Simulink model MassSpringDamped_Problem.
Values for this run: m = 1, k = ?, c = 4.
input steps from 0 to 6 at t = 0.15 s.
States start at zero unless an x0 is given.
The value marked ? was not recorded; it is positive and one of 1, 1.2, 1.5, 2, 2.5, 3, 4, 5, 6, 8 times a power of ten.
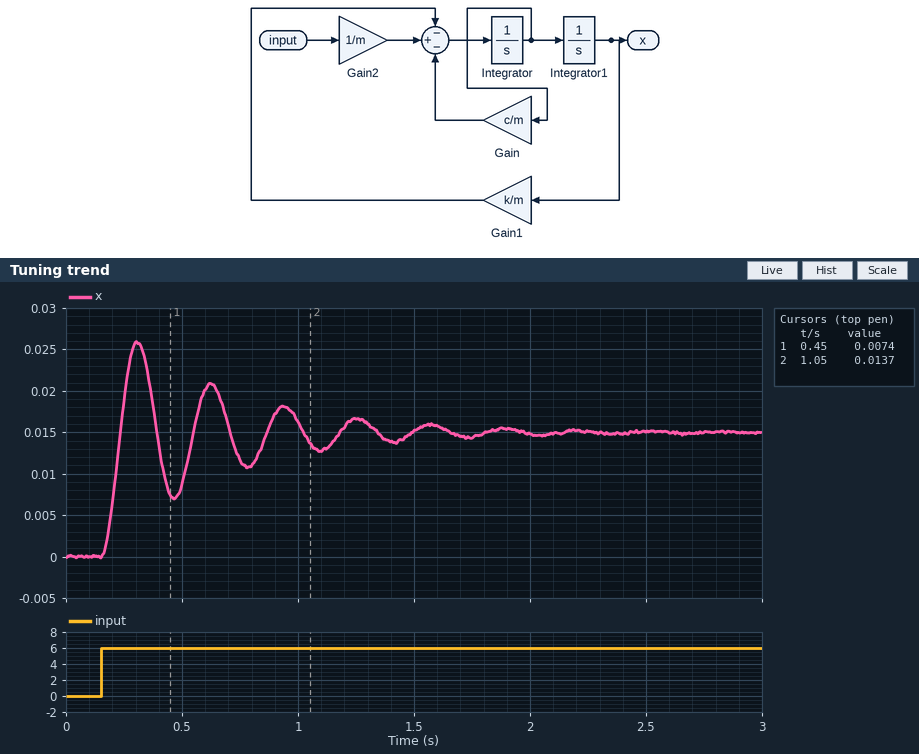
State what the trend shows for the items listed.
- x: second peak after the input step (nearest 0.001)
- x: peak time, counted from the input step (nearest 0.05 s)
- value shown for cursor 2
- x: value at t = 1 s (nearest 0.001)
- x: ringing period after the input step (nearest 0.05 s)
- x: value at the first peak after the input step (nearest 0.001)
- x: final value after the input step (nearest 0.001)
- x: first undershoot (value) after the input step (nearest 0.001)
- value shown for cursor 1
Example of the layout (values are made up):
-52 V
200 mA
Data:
0.021
0.15 s
0.0137
0.016
0.30 s
0.026
0.015
0.007
0.0074
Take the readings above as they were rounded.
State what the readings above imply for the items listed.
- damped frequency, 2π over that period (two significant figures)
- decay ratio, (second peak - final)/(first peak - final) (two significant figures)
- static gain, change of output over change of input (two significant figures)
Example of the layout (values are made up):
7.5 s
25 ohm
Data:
21 rad/s
0.55
0.0025
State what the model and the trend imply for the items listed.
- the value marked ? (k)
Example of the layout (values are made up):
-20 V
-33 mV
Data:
400
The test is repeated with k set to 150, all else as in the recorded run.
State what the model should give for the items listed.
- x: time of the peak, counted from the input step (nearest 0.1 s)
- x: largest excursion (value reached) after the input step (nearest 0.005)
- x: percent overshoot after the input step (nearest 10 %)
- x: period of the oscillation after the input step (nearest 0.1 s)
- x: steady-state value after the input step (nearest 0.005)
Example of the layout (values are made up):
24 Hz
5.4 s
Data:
0.3 s
0.065
60 %
0.5 s
0.040
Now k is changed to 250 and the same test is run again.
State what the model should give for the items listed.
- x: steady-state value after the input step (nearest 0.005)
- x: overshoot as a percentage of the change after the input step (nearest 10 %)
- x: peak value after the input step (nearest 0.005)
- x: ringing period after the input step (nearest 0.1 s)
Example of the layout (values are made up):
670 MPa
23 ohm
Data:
0.025
70 %
0.040
0.4 s
